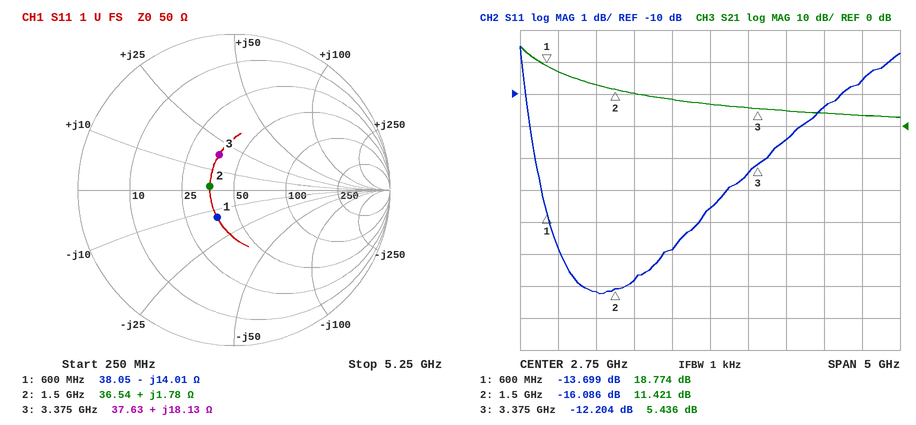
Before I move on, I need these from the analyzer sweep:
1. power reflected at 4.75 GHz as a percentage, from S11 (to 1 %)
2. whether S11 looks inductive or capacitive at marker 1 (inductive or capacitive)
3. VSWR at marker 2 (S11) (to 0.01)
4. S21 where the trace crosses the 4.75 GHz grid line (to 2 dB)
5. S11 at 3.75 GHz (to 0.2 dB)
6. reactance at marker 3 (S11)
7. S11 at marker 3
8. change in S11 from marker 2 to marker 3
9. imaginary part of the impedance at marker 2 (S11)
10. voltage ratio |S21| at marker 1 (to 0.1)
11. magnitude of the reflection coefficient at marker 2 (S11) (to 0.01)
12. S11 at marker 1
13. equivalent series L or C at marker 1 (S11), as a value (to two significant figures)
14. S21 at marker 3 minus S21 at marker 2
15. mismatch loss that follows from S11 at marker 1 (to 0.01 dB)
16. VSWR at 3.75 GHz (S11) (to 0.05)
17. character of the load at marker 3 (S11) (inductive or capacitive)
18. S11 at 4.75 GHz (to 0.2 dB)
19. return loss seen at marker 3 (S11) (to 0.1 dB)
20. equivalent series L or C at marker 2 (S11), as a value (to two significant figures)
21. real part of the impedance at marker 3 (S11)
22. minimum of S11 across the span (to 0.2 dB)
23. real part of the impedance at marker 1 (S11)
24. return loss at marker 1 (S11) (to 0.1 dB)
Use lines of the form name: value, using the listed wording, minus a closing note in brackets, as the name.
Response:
power reflected at 4.75 GHz as a percentage, from S11: 11 %
whether S11 looks inductive or capacitive at marker 1: capacitive
VSWR at marker 2 (S11): 1.37
S21 where the trace crosses the 4.75 GHz grid line: 4 dB
S11 at 3.75 GHz: -11.4 dB
reactance at marker 3: +18.13 Ω
S11 at marker 3: -12.204 dB
change in S11 from marker 2 to marker 3: 3.882 dB
imaginary part of the impedance at marker 2: +1.78 Ω
voltage ratio |S21| at marker 1: 8.7
magnitude of the reflection coefficient at marker 2 (S11): 0.16
S11 at marker 1: -13.699 dB
equivalent series L or C at marker 1 (S11), as a value: 19 pF
S21 at marker 3 minus S21 at marker 2: -5.985 dB
mismatch loss that follows from S11 at marker 1: 0.19 dB
VSWR at 3.75 GHz (S11): 1.75
character of the load at marker 3 (S11): inductive
S11 at 4.75 GHz: -9.6 dB
return loss seen at marker 3 (S11): 12.2 dB
equivalent series L or C at marker 2 (S11), as a value: 190 pH
real part of the impedance at marker 3: 37.63 Ω
minimum of S11 across the span: -16.2 dB
real part of the impedance at marker 1: 38.05 Ω
return loss at marker 1 (S11): 13.7 dB
